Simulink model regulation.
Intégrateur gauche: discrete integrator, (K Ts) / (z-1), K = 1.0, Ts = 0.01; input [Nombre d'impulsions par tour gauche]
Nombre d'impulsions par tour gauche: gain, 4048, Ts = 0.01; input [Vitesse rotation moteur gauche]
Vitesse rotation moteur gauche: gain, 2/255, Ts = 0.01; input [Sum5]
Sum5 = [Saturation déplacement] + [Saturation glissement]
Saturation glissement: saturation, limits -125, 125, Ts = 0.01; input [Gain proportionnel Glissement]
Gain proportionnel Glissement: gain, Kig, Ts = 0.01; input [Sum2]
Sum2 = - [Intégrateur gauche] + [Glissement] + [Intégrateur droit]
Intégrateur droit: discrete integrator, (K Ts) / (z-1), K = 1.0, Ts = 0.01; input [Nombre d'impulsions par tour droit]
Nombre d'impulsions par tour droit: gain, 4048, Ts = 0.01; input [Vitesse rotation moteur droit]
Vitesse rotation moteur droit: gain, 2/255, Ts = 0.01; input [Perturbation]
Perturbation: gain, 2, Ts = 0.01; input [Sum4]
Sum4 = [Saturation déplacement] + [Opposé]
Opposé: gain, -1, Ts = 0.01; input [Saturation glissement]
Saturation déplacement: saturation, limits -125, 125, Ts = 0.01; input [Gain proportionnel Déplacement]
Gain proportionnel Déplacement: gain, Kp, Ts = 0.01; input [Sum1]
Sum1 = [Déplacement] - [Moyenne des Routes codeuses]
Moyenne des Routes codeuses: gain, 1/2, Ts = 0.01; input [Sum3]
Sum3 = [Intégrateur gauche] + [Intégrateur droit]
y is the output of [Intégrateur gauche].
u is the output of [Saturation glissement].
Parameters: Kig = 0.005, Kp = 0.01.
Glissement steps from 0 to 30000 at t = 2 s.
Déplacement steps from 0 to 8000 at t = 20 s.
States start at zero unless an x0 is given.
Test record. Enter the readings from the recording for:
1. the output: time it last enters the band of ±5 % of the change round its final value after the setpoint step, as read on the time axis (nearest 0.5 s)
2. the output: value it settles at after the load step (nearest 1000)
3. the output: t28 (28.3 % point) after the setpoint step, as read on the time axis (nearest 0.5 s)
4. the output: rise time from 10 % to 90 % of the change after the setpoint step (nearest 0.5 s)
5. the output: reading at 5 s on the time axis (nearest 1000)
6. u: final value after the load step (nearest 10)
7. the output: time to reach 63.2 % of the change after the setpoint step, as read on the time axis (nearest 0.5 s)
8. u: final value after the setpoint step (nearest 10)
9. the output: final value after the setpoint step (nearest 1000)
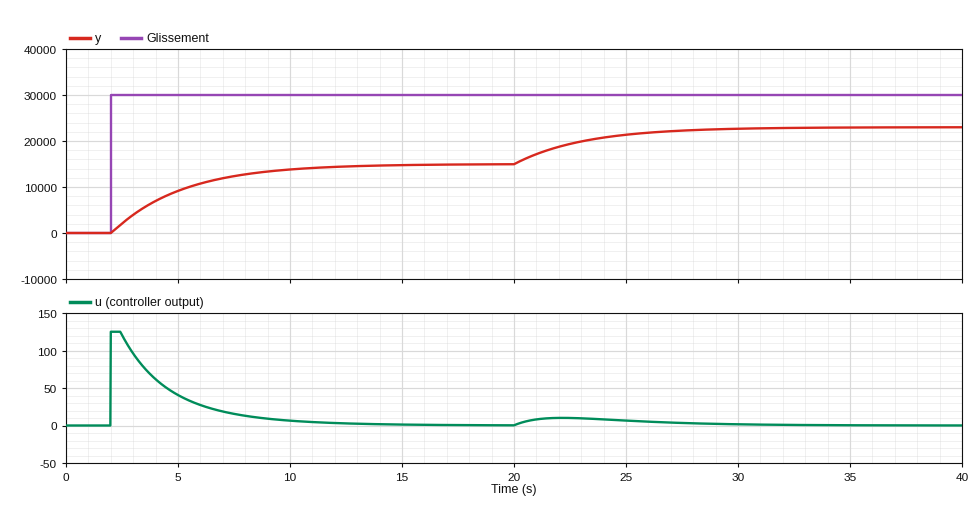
11.5 s
23000
3.0 s
7.0 s
9000
0
5.0 s
0
15000
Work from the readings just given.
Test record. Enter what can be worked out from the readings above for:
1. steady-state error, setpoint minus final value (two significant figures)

15000
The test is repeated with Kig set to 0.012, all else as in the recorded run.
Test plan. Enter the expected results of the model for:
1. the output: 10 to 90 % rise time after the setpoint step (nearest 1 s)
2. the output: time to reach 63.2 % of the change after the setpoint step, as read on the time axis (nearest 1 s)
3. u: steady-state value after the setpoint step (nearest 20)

5 s
4 s
0
